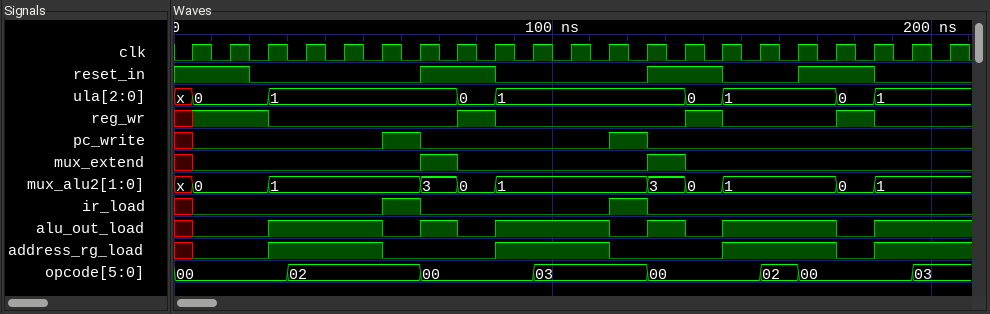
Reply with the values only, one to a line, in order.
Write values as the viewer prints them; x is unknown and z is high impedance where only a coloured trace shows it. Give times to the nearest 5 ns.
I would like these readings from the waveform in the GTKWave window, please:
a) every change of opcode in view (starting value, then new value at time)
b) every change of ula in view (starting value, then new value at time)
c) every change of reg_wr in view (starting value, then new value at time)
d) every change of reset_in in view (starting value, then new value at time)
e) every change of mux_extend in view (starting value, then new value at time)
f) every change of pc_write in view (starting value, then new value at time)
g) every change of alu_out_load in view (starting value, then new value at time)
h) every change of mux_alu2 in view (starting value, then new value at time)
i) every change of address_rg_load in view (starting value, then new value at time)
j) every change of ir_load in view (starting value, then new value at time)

00, 02 at 30 ns, 00 at 65 ns, 03 at 95 ns, 00 at 125 ns, 02 at 155 ns, 00 at 165 ns, 03 at 195 ns
x, 0 at 5 ns, 1 at 25 ns, 0 at 75 ns, 1 at 85 ns, 0 at 135 ns, 1 at 145 ns, 0 at 175 ns, 1 at 185 ns
x, 1 at 5 ns, 0 at 25 ns, 1 at 75 ns, 0 at 85 ns, 1 at 135 ns, 0 at 145 ns, 1 at 175 ns, 0 at 185 ns
1, 0 at 20 ns, 1 at 65 ns, 0 at 85 ns, 1 at 125 ns, 0 at 145 ns, 1 at 165 ns, 0 at 185 ns
x, 0 at 5 ns, 1 at 65 ns, 0 at 75 ns, 1 at 125 ns, 0 at 135 ns
x, 0 at 5 ns, 1 at 55 ns, 0 at 65 ns, 1 at 115 ns, 0 at 125 ns
x, 0 at 5 ns, 1 at 25 ns, 0 at 55 ns, 1 at 65 ns, 0 at 75 ns, 1 at 85 ns, 0 at 115 ns, 1 at 125 ns, 0 at 135 ns, 1 at 145 ns, 0 at 175 ns, 1 at 185 ns
x, 0 at 5 ns, 1 at 25 ns, 3 at 65 ns, 0 at 75 ns, 1 at 85 ns, 3 at 125 ns, 0 at 135 ns, 1 at 145 ns, 0 at 175 ns, 1 at 185 ns
x, 0 at 5 ns, 1 at 25 ns, 0 at 55 ns, 1 at 85 ns, 0 at 115 ns, 1 at 145 ns, 0 at 175 ns, 1 at 185 ns
x, 0 at 5 ns, 1 at 55 ns, 0 at 65 ns, 1 at 115 ns, 0 at 125 ns
